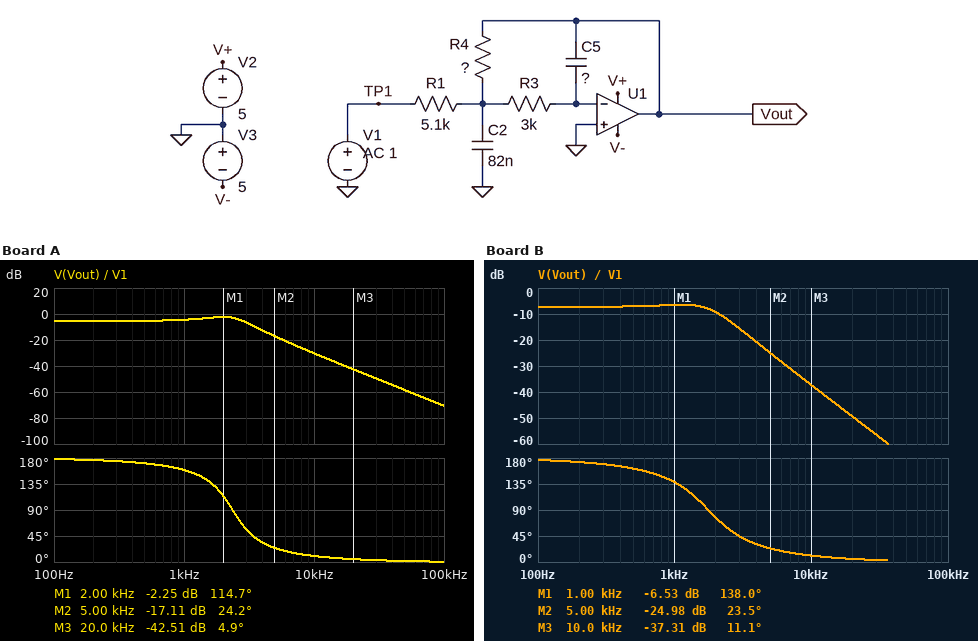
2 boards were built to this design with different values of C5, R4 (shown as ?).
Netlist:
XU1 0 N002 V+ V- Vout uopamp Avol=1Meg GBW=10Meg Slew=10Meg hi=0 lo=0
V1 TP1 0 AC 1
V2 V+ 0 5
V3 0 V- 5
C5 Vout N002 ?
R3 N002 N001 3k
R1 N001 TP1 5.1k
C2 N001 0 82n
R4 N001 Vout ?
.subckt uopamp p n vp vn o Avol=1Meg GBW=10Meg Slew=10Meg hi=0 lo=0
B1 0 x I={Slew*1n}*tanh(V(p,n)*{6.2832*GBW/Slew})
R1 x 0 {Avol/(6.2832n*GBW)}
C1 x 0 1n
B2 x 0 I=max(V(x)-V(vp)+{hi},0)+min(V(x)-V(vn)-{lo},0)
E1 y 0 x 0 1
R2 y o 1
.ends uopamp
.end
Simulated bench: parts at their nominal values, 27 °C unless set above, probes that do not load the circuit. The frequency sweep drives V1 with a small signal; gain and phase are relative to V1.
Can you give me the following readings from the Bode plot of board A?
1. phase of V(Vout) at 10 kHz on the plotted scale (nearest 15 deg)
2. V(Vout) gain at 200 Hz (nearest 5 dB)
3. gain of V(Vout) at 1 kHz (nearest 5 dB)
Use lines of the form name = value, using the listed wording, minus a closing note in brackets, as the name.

phase of V(Vout) at 10 kHz on the plotted scale = 15 deg
V(Vout) gain at 200 Hz = -5 dB
gain of V(Vout) at 1 kHz = -5 dB
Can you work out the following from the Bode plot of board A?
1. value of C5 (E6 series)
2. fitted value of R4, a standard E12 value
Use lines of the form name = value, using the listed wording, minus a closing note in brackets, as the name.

value of C5 = 6.8 nF
fitted value of R4, a standard E12 value = 2.7 kΩ
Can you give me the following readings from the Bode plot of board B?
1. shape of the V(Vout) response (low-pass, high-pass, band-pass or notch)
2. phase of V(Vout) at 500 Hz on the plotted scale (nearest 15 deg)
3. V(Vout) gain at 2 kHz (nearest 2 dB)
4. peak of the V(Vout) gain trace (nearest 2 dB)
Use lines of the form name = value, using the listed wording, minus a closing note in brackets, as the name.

shape of the V(Vout) response = low-pass
phase of V(Vout) at 500 Hz on the plotted scale = 165 deg
V(Vout) gain at 2 kHz = -10 dB
peak of the V(Vout) gain trace = -6 dB
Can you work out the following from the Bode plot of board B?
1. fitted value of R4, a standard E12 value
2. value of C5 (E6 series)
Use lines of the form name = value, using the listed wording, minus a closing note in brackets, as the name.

fitted value of R4, a standard E12 value = 2.2 kΩ
value of C5 = 15 nF
